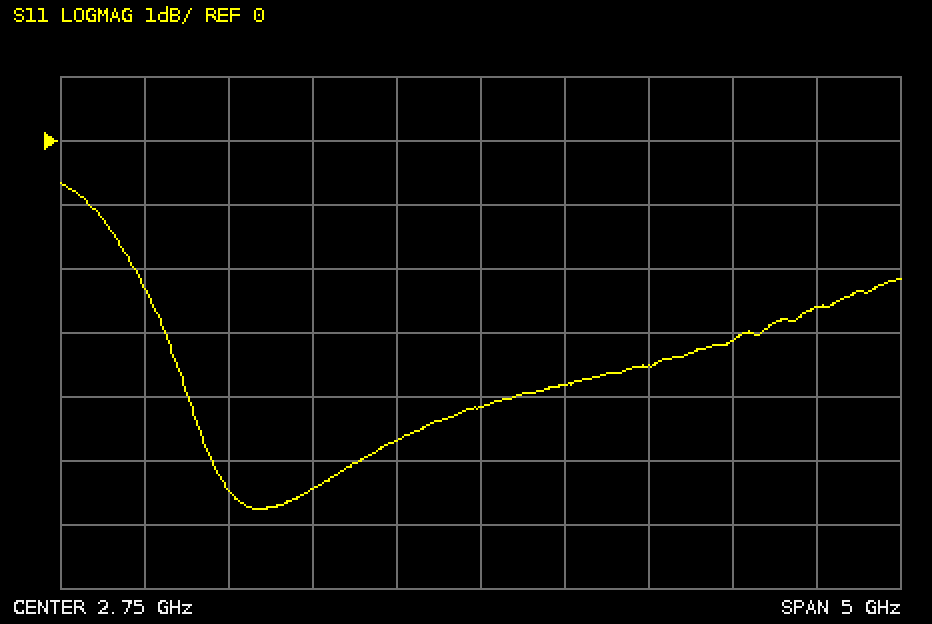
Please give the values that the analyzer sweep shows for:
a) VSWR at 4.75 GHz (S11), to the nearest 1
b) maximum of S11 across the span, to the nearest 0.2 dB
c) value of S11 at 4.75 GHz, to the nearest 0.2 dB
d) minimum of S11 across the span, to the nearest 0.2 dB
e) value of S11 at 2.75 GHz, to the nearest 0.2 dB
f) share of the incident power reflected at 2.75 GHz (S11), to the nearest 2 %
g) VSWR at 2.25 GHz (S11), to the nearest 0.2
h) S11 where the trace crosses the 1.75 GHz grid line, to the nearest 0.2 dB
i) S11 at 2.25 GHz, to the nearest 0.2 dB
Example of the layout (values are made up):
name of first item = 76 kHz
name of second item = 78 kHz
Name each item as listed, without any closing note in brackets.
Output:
VSWR at 4.75 GHz (S11), to the nearest 1 = 7
maximum of S11 across the span, to the nearest 0.2 dB = -0.6 dB
value of S11 at 4.75 GHz, to the nearest 0.2 dB = -2.6 dB
minimum of S11 across the span, to the nearest 0.2 dB = -5.8 dB
value of S11 at 2.75 GHz, to the nearest 0.2 dB = -4.2 dB
share of the incident power reflected at 2.75 GHz (S11), to the nearest 2 % = 38 %
VSWR at 2.25 GHz (S11), to the nearest 0.2 = 3.8
S11 where the trace crosses the 1.75 GHz grid line, to the nearest 0.2 dB = -5.4 dB
S11 at 2.25 GHz, to the nearest 0.2 dB = -4.6 dB
